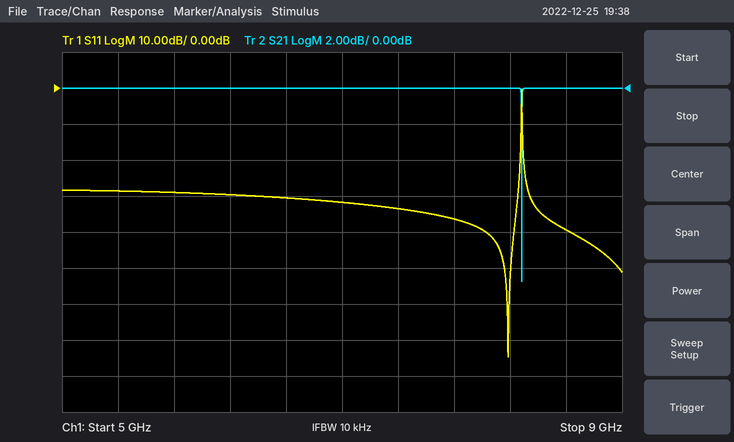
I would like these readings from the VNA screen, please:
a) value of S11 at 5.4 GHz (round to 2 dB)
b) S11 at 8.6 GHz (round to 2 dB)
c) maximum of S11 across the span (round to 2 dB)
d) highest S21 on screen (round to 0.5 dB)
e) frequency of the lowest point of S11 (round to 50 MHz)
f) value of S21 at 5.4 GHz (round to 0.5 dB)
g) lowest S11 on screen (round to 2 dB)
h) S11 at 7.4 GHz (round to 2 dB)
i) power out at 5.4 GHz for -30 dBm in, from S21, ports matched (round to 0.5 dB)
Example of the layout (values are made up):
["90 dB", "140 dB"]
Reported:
["-28 dB", "-40 dB", "0 dB", "0.0 dB", "8.20 GHz", "0.0 dB", "-74 dB", "-34 dB", "-30.0 dBm"]
